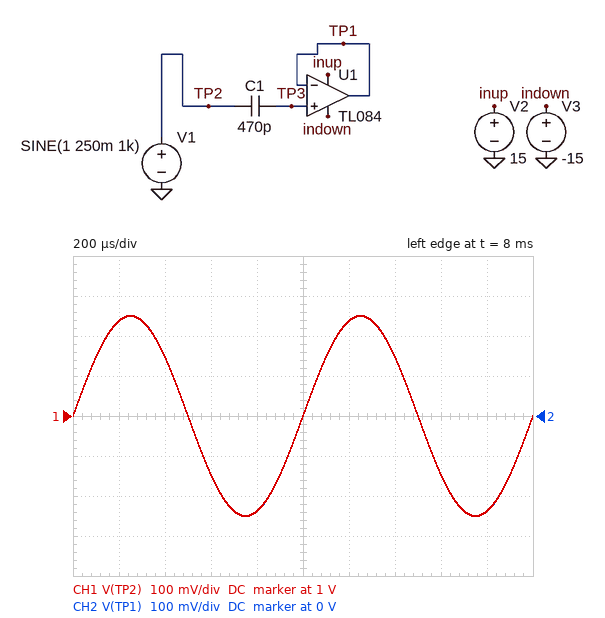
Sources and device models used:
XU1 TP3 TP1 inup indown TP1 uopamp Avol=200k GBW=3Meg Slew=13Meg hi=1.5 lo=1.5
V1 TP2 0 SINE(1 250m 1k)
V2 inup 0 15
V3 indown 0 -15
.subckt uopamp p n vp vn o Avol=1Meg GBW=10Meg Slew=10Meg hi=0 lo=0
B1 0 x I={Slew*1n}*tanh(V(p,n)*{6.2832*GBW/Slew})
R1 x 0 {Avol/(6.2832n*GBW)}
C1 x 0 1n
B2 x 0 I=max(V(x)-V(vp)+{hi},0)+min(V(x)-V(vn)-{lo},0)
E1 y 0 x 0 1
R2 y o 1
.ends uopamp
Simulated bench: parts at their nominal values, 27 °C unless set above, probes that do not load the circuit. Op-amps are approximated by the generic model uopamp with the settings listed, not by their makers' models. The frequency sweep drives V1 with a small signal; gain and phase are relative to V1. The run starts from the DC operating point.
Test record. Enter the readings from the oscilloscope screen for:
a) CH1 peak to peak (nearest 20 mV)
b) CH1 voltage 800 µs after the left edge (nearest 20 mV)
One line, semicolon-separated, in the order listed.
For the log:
500 mV; 760 mV
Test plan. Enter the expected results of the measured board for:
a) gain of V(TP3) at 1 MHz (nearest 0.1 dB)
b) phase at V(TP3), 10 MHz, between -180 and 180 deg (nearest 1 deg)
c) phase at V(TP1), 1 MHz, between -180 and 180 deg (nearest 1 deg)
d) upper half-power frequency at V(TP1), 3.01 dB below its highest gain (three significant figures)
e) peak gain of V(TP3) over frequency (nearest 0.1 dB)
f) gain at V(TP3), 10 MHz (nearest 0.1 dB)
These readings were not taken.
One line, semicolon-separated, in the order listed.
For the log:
0 dB; 0 deg; -18 deg; 3.00 MHz; 0 dB; 0 dB
